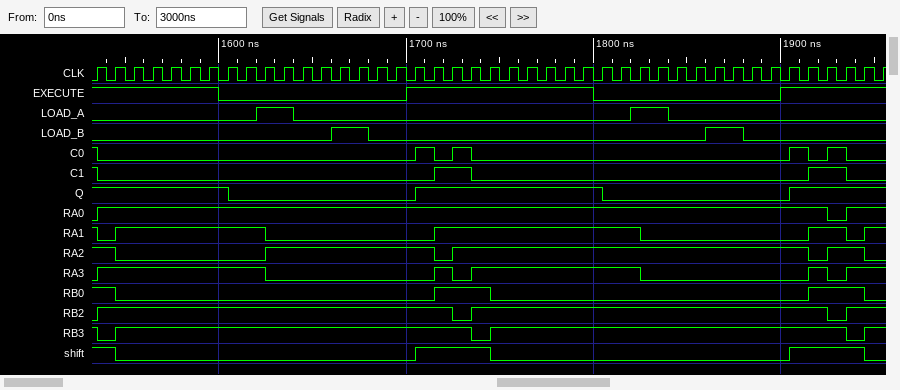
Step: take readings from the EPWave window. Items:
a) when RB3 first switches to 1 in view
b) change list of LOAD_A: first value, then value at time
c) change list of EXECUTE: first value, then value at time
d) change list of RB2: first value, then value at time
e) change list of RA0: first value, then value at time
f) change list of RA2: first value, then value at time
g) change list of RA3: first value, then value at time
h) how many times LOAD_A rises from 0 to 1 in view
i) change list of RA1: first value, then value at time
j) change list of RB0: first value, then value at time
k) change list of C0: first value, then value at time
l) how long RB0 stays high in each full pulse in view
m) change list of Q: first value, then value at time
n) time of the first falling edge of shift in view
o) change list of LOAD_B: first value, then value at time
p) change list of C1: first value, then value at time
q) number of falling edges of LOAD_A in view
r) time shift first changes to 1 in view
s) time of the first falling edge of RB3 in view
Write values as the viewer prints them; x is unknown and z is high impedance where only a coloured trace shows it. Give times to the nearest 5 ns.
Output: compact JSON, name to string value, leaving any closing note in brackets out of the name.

{"when RB3 first switches to 1 in view": "1545 ns", "change list of LOAD_A: first value, then value at time": "0, 1 at 1620 ns, 0 at 1640 ns, 1 at 1820 ns, 0 at 1840 ns", "change list of EXECUTE: first value, then value at time": "1, 0 at 1600 ns, 1 at 1700 ns, 0 at 1800 ns, 1 at 1900 ns", "change list of RB2: first value, then value at time": "0, 1 at 1535 ns, 0 at 1725 ns, 1 at 1735 ns, 0 at 1925 ns, 1 at 1935 ns", "change list of RA0: first value, then value at time": "0, 1 at 1535 ns, 0 at 1925 ns, 1 at 1935 ns", "change list of RA2: first value, then value at time": "1, 0 at 1545 ns, 1 at 1625 ns, 0 at 1715 ns, 1 at 1725 ns, 0 at 1915 ns, 1 at 1925 ns, 0 at 1945 ns", "change list of RA3: first value, then value at time": "0, 1 at 1535 ns, 0 at 1625 ns, 1 at 1715 ns, 0 at 1725 ns, 1 at 1735 ns, 0 at 1825 ns, 1 at 1915 ns, 0 at 1925 ns, 1 at 1935 ns", "how many times LOAD_A rises from 0 to 1 in view": "2", "change list of RA1: first value, then value at time": "1, 0 at 1535 ns, 1 at 1545 ns, 0 at 1625 ns, 1 at 1715 ns, 0 at 1825 ns, 1 at 1915 ns, 0 at 1935 ns, 1 at 1945 ns", "change list of RB0: first value, then value at time": "1, 0 at 1545 ns, 1 at 1715 ns, 0 at 1745 ns, 1 at 1915 ns, 0 at 1945 ns", "change list of C0: first value, then value at time": "1, 0 at 1535 ns, 1 at 1705 ns, 0 at 1715 ns, 1 at 1725 ns, 0 at 1735 ns, 1 at 1905 ns, 0 at 1915 ns, 1 at 1925 ns, 0 at 1935 ns", "how long RB0 stays high in each full pulse in view": "30 ns, 30 ns", "change list of Q: first value, then value at time": "1, 0 at 1605 ns, 1 at 1705 ns, 0 at 1805 ns, 1 at 1905 ns", "time of the first falling edge of shift in view": "1545 ns", "change list of LOAD_B: first value, then value at time": "0, 1 at 1660 ns, 0 at 1680 ns, 1 at 1860 ns, 0 at 1880 ns", "change list of C1: first value, then value at time": "1, 0 at 1535 ns, 1 at 1715 ns, 0 at 1735 ns, 1 at 1915 ns, 0 at 1935 ns", "number of falling edges of LOAD_A in view": "2", "time shift first changes to 1 in view": "1705 ns", "time of the first falling edge of RB3 in view": "1535 ns"}
